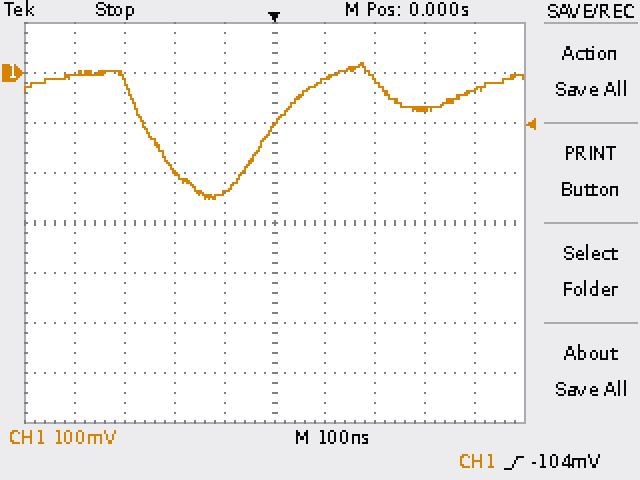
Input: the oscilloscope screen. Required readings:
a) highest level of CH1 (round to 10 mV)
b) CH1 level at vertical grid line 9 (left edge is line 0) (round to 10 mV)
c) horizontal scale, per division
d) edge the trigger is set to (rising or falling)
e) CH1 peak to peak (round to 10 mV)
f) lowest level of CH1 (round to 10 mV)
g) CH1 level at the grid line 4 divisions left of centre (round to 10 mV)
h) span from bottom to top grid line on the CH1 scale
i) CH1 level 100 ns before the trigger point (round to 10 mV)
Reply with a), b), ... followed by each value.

a) 20 mV
b) -30 mV
c) 100 ns
d) rising
e) 270 mV
f) -250 mV
g) 0 mV
h) 800 mV
i) -240 mV
